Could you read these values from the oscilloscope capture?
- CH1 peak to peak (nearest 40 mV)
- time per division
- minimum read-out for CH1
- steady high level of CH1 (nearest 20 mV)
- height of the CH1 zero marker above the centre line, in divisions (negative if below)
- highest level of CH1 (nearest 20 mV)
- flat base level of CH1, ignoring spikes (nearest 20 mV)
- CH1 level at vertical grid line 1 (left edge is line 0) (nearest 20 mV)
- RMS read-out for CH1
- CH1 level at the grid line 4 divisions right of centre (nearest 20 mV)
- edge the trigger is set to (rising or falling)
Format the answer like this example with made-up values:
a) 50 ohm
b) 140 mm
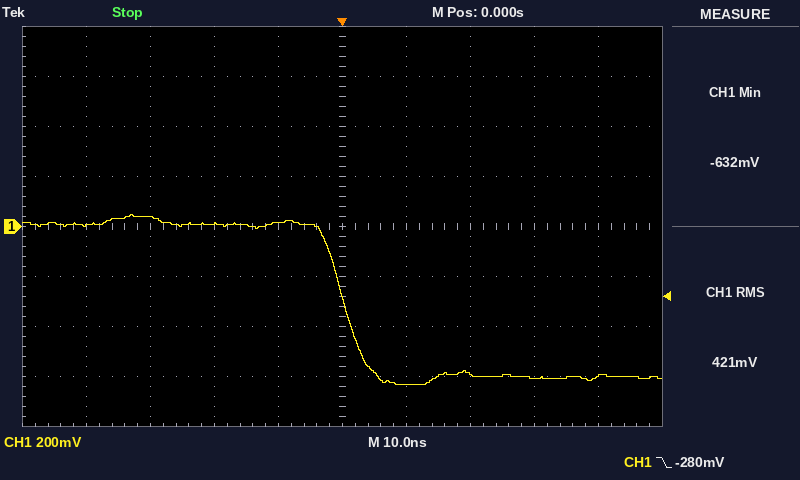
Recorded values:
a) 680 mV
b) 10 ns
c) -632 mV
d) 0 mV
e) 0.0 div
f) 40 mV
g) -600 mV
h) 0 mV
i) 421 mV
j) -600 mV
k) falling
